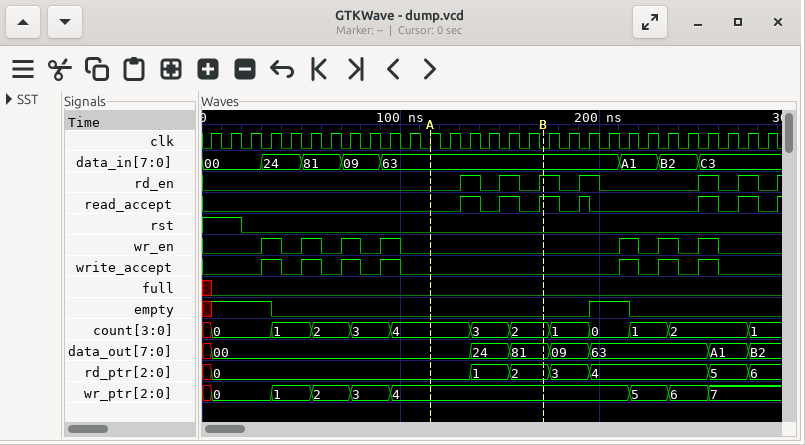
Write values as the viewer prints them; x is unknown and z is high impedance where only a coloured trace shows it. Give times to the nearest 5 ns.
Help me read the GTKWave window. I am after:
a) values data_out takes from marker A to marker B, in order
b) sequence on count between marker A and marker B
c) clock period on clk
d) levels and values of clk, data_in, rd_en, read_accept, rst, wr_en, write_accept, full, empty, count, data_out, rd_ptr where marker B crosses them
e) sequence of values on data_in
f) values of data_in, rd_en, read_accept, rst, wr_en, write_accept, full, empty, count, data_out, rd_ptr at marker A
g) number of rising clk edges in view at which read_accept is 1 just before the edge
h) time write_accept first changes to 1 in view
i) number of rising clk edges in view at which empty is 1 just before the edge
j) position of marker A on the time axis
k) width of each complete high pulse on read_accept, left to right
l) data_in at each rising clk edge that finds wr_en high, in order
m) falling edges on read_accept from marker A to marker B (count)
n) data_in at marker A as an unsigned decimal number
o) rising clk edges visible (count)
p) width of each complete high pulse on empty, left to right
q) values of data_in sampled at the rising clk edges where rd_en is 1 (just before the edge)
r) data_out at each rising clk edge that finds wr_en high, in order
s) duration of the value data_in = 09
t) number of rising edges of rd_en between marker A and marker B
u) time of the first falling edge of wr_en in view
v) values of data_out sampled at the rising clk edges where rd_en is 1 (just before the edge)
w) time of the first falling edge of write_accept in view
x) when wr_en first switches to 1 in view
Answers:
00, 24, 81
4, 3, 2
10 ns
clk=0, data_in=63, rd_en=1, read_accept=1, rst=0, wr_en=0, write_accept=0, full=0, empty=0, count=2, data_out=81, rd_ptr=2
00, 24, 81, 09, 63, A1, B2, C3
data_in=63, rd_en=0, read_accept=0, rst=0, wr_en=0, write_accept=0, full=0, empty=0, count=4, data_out=00, rd_ptr=0
6
30 ns
5
115 ns
10 ns, 10 ns, 10 ns, 5 ns, 10 ns, 10 ns
24, 81, 09, 63, A1, B2, C3
2
99
29
20 ns
63, 63, 63, 63, C3, C3
00, 00, 00, 00, 63, 63, 63
20 ns
3
40 ns
00, 24, 81, 09, 63, A1
40 ns
30 ns
